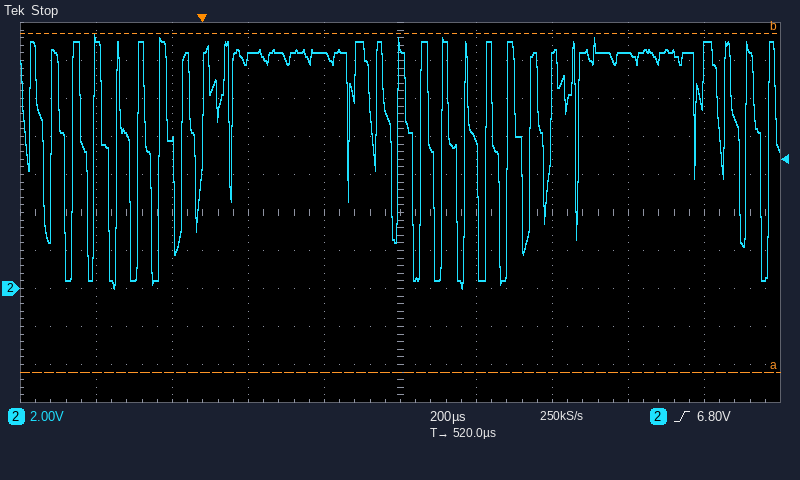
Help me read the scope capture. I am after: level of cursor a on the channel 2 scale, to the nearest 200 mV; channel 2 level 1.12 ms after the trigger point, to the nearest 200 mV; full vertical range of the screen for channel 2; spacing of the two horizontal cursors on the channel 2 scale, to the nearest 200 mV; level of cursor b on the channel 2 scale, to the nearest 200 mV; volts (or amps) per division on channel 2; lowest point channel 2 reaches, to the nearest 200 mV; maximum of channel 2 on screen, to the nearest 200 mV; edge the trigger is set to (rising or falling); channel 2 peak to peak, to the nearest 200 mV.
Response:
-4.4 V
12.4 V
20 V
17.8 V
13.4 V
2 V
0.0 V
13.4 V
rising
13.4 V
